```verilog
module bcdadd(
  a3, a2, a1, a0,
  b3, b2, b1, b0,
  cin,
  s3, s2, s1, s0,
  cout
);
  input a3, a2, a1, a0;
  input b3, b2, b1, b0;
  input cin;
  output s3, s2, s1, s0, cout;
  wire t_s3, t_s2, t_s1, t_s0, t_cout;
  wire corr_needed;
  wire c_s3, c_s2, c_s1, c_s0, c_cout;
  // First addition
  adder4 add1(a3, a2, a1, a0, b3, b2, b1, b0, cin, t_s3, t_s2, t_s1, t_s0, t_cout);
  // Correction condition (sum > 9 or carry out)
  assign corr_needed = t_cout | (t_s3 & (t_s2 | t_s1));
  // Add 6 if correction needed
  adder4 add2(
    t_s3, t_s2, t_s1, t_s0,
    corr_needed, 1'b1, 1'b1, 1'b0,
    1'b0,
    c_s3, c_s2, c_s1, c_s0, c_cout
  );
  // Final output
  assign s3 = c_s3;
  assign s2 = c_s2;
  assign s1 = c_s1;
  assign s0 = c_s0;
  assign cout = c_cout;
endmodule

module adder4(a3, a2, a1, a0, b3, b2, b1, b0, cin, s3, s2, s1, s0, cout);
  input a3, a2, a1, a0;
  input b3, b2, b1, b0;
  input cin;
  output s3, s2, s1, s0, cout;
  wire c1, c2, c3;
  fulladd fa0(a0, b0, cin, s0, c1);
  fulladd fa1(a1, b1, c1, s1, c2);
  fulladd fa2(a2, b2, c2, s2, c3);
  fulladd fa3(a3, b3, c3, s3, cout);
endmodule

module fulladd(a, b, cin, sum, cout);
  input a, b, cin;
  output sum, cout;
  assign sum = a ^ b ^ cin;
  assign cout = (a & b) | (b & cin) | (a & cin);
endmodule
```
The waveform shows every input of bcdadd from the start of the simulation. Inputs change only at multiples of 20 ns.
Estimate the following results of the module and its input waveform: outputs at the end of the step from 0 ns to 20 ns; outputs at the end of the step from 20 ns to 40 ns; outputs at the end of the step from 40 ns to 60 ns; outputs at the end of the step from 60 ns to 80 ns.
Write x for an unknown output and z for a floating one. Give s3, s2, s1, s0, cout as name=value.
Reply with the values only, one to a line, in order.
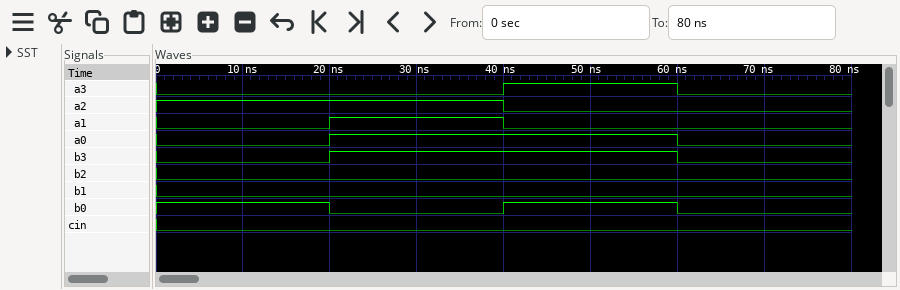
s3=1, s2=0, s1=1, s0=1, cout=0
s3=1, s2=1, s1=0, s0=1, cout=1
s3=0, s2=0, s1=0, s0=0, cout=1
s3=0, s2=1, s1=1, s0=0, cout=0
